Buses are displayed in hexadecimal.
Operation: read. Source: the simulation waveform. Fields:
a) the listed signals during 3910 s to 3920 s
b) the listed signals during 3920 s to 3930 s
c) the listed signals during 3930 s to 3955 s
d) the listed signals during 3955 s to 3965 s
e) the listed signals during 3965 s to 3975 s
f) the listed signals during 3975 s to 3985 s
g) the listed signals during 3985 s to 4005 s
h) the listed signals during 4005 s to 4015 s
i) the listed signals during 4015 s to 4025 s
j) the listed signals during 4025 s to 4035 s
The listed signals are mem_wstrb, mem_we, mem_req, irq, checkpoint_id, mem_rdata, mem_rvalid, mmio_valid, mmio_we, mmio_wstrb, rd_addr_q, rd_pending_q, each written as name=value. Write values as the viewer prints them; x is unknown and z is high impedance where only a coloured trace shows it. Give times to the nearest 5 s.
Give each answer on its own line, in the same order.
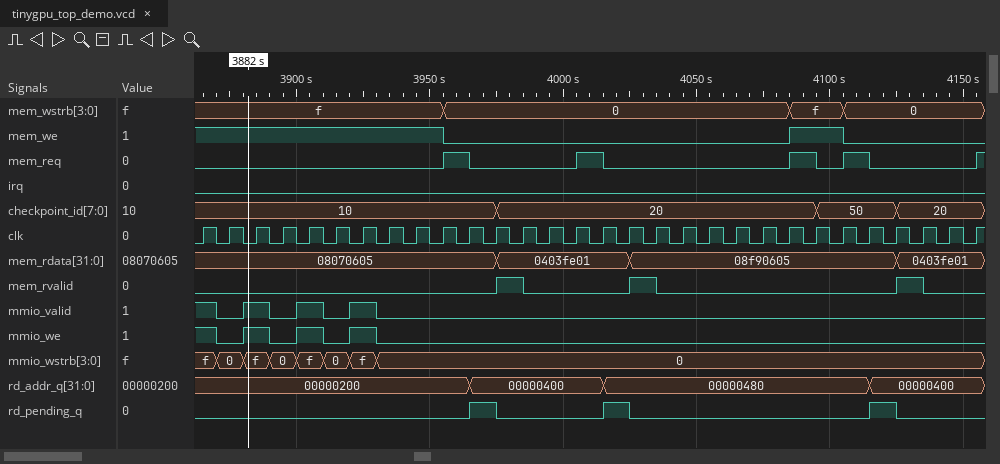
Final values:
mem_wstrb=f, mem_we=1, mem_req=0, irq=0, checkpoint_id=10, mem_rdata=08070605, mem_rvalid=0, mmio_valid=0, mmio_we=0, mmio_wstrb=0, rd_addr_q=00000200, rd_pending_q=0
mem_wstrb=f, mem_we=1, mem_req=0, irq=0, checkpoint_id=10, mem_rdata=08070605, mem_rvalid=0, mmio_valid=1, mmio_we=1, mmio_wstrb=f, rd_addr_q=00000200, rd_pending_q=0
mem_wstrb=f, mem_we=1, mem_req=0, irq=0, checkpoint_id=10, mem_rdata=08070605, mem_rvalid=0, mmio_valid=0, mmio_we=0, mmio_wstrb=0, rd_addr_q=00000200, rd_pending_q=0
mem_wstrb=0, mem_we=0, mem_req=1, irq=0, checkpoint_id=10, mem_rdata=08070605, mem_rvalid=0, mmio_valid=0, mmio_we=0, mmio_wstrb=0, rd_addr_q=00000200, rd_pending_q=0
mem_wstrb=0, mem_we=0, mem_req=0, irq=0, checkpoint_id=10, mem_rdata=08070605, mem_rvalid=0, mmio_valid=0, mmio_we=0, mmio_wstrb=0, rd_addr_q=00000400, rd_pending_q=1
mem_wstrb=0, mem_we=0, mem_req=0, irq=0, checkpoint_id=20, mem_rdata=0403fe01, mem_rvalid=1, mmio_valid=0, mmio_we=0, mmio_wstrb=0, rd_addr_q=00000400, rd_pending_q=0
mem_wstrb=0, mem_we=0, mem_req=0, irq=0, checkpoint_id=20, mem_rdata=0403fe01, mem_rvalid=0, mmio_valid=0, mmio_we=0, mmio_wstrb=0, rd_addr_q=00000400, rd_pending_q=0
mem_wstrb=0, mem_we=0, mem_req=1, irq=0, checkpoint_id=20, mem_rdata=0403fe01, mem_rvalid=0, mmio_valid=0, mmio_we=0, mmio_wstrb=0, rd_addr_q=00000400, rd_pending_q=0
mem_wstrb=0, mem_we=0, mem_req=0, irq=0, checkpoint_id=20, mem_rdata=0403fe01, mem_rvalid=0, mmio_valid=0, mmio_we=0, mmio_wstrb=0, rd_addr_q=00000480, rd_pending_q=1
mem_wstrb=0, mem_we=0, mem_req=0, irq=0, checkpoint_id=20, mem_rdata=08f90605, mem_rvalid=1, mmio_valid=0, mmio_we=0, mmio_wstrb=0, rd_addr_q=00000480, rd_pending_q=0
